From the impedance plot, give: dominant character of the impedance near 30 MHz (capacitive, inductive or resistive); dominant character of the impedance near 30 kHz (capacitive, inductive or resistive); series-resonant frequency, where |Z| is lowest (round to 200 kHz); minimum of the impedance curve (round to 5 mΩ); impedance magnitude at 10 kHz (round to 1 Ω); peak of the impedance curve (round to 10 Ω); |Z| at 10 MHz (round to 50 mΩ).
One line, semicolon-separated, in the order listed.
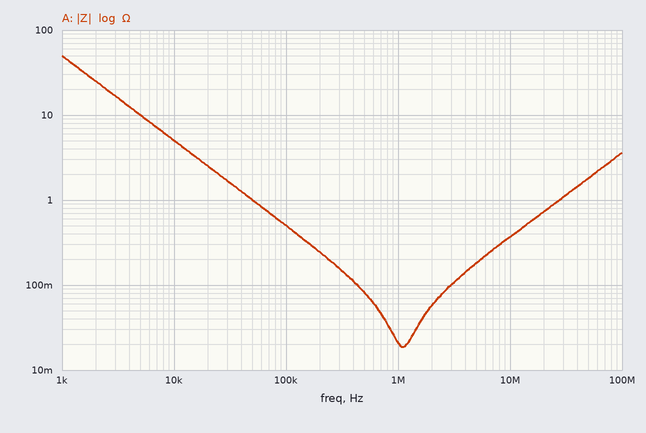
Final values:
inductive; capacitive; 1.2 MHz; 20 mΩ; 5 Ω; 50 Ω; 350 mΩ
